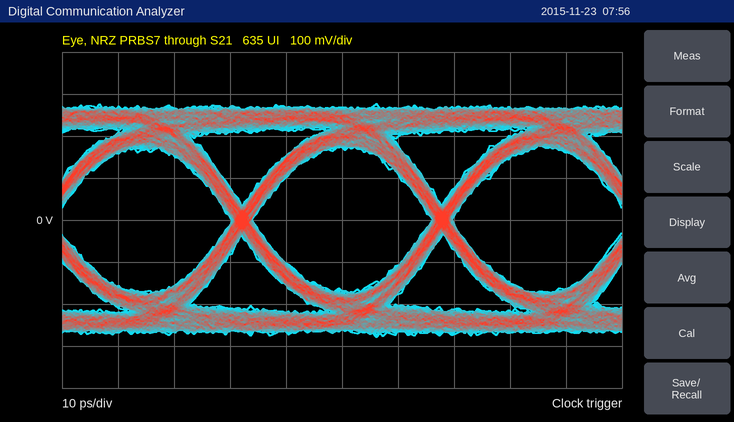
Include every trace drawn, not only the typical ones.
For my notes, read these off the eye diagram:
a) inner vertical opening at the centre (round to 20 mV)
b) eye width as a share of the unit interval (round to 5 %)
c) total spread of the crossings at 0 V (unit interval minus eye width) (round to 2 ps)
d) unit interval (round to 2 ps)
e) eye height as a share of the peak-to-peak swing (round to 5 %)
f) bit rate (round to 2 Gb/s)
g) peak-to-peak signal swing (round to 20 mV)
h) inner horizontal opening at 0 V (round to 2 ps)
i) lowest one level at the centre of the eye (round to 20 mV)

340 mV
90 %
4 ps
36 ps
60 %
28 Gb/s
560 mV
32 ps
180 mV
